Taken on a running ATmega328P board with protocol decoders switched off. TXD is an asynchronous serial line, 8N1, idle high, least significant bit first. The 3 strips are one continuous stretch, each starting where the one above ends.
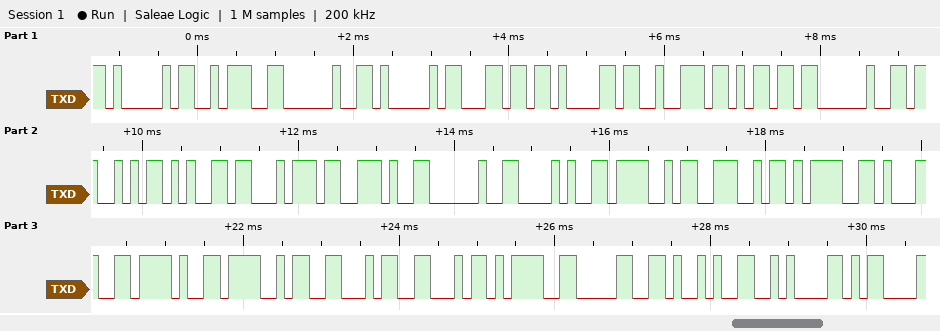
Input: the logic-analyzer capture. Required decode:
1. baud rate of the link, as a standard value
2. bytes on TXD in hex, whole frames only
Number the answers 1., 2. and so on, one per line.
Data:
1. 9600 baud
2. 41 3A 20 41 6C 61 72 6D 20 53 65 74 2E 20 28 4F 4E 3D 31 2F 4F 46 46 3D 30 29 0A 0D
